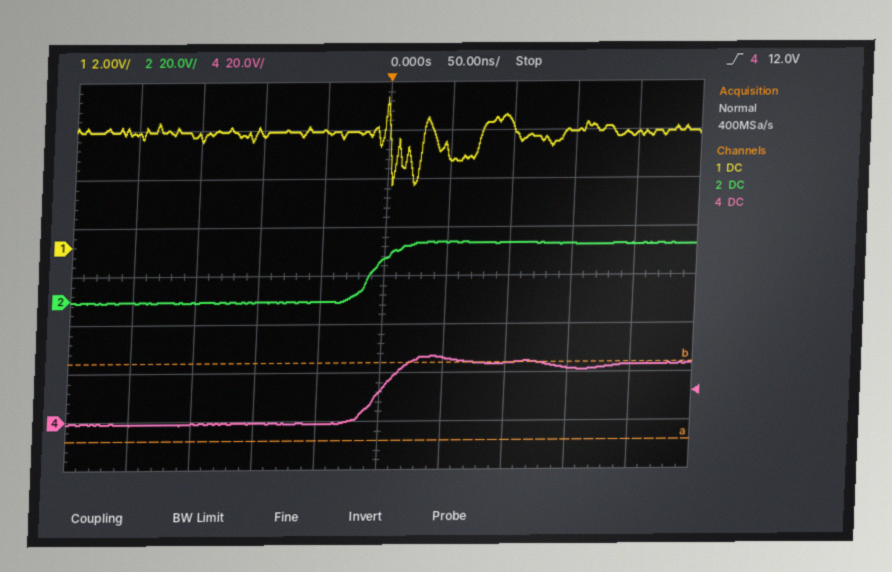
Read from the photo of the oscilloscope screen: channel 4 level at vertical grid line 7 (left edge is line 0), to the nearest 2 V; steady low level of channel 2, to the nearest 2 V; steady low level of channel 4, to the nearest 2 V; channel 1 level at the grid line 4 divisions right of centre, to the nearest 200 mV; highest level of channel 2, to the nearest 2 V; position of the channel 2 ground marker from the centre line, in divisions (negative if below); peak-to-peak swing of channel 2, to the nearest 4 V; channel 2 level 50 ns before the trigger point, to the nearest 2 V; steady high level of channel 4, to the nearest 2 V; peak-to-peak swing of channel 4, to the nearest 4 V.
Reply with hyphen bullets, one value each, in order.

- 24 V
- 0 V
- 0 V
- 4.6 V
- 24 V
- -0.5 div
- 24 V
- 0 V
- 24 V
- 28 V
